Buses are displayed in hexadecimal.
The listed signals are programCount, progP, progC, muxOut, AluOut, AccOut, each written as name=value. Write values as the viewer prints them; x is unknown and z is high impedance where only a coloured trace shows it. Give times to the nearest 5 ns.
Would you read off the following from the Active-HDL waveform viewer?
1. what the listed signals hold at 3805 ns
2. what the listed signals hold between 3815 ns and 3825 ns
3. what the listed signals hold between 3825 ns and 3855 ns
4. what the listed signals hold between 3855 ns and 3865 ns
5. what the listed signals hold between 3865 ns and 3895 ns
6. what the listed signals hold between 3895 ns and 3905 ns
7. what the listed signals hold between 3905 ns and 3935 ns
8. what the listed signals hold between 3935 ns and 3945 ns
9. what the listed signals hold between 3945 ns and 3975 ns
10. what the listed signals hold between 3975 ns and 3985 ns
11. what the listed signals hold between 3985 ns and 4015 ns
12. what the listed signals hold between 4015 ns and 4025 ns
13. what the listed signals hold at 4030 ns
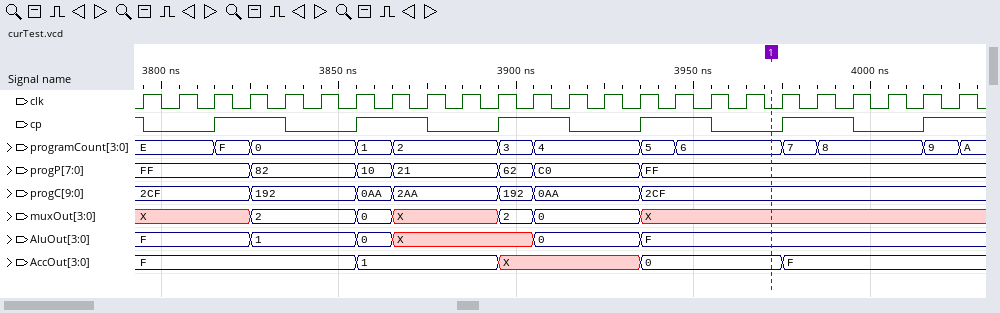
programCount=E, progP=FF, progC=2CF, muxOut=X, AluOut=F, AccOut=F
programCount=F, progP=FF, progC=2CF, muxOut=X, AluOut=F, AccOut=F
programCount=0, progP=82, progC=192, muxOut=2, AluOut=1, AccOut=F
programCount=1, progP=10, progC=0AA, muxOut=0, AluOut=0, AccOut=1
programCount=2, progP=21, progC=2AA, muxOut=X, AluOut=X, AccOut=1
programCount=3, progP=62, progC=192, muxOut=2, AluOut=X, AccOut=X
programCount=4, progP=C0, progC=0AA, muxOut=0, AluOut=0, AccOut=X
programCount=5, progP=FF, progC=2CF, muxOut=X, AluOut=F, AccOut=0
programCount=6, progP=FF, progC=2CF, muxOut=X, AluOut=F, AccOut=0
programCount=7, progP=FF, progC=2CF, muxOut=X, AluOut=F, AccOut=F
programCount=8, progP=FF, progC=2CF, muxOut=X, AluOut=F, AccOut=F
programCount=9, progP=FF, progC=2CF, muxOut=X, AluOut=F, AccOut=F
programCount=A, progP=FF, progC=2CF, muxOut=X, AluOut=F, AccOut=F
